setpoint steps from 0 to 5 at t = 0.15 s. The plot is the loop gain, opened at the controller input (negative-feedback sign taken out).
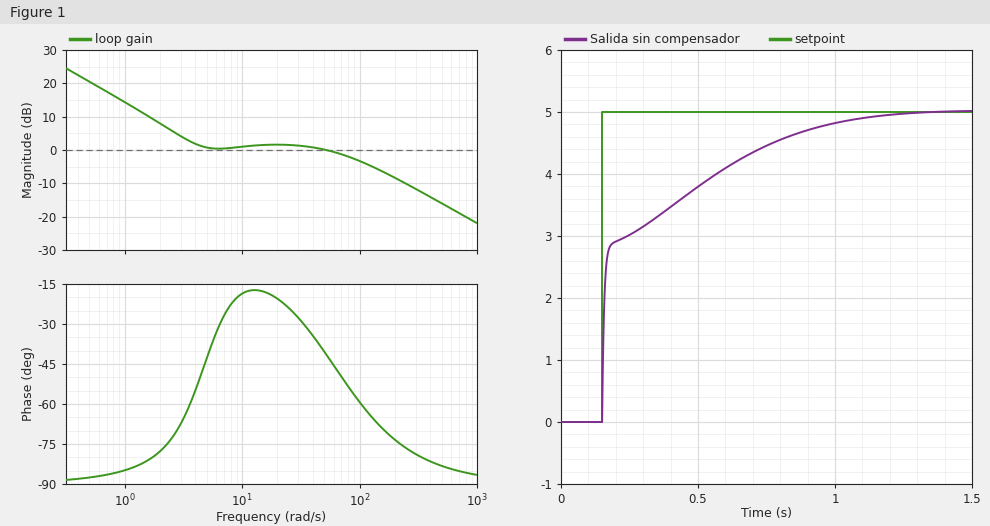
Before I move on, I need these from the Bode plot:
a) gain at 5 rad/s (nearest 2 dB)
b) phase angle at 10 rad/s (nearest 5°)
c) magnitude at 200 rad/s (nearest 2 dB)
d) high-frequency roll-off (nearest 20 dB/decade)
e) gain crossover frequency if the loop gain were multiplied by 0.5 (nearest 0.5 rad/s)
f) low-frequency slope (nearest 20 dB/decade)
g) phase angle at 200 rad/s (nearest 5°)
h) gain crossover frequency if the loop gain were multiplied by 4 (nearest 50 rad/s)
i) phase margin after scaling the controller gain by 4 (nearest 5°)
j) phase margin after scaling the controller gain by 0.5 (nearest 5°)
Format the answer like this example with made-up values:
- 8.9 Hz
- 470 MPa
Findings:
- 0 dB
- -20°
- -8 dB
- -20 dB/decade
- 2.5 rad/s
- -20 dB/decade
- -75°
- 300 rad/s
- 100°
- 105°
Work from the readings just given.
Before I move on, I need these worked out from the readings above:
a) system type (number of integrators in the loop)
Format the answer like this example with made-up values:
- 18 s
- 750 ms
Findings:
- 1
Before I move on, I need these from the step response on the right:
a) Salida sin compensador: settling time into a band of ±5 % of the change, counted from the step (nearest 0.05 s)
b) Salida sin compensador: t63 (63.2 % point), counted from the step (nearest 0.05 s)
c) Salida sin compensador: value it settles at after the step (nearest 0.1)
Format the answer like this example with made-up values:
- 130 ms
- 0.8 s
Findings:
- 0.80 s
- 0.15 s
- 5.0
